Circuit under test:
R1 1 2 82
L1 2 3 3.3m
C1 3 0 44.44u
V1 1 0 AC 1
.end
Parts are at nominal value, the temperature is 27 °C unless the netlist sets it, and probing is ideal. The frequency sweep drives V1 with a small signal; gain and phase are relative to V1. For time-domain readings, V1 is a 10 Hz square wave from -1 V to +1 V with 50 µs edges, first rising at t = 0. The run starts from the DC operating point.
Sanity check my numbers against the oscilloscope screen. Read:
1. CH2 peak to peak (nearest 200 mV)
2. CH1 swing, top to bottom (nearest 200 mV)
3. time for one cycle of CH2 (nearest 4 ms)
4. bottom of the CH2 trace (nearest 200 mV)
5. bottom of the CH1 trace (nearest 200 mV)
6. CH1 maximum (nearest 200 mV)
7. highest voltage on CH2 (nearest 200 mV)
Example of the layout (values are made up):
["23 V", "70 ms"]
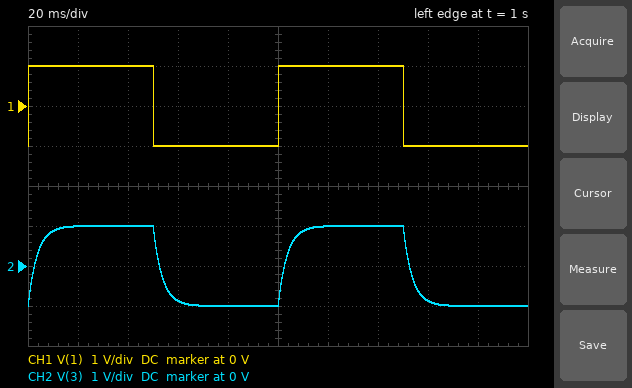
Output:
["2.0 V", "2.0 V", "100 ms", "-1.0 V", "-1.0 V", "1.0 V", "1.0 V"]
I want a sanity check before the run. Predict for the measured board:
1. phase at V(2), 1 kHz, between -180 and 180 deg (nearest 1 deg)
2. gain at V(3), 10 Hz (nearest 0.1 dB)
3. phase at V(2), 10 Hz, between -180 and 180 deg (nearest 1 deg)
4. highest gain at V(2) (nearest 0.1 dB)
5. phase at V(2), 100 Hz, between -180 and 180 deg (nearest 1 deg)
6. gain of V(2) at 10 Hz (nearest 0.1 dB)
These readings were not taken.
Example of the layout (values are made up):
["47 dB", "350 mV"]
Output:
["78 deg", "-0.2 dB", "-13 deg", "0 dB", "-68 deg", "-0.2 dB"]
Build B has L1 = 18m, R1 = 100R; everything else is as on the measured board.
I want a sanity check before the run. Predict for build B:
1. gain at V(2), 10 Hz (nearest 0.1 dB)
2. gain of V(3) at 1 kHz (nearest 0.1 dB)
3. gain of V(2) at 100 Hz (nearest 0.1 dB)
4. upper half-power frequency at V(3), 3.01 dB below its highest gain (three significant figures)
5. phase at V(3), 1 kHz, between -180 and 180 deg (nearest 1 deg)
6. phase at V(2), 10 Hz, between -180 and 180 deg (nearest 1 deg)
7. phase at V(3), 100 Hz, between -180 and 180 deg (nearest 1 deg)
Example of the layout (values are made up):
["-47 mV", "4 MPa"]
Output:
["-0.3 dB", "-32.3 dB", "-12.5 dB", "37.3 Hz", "-138 deg", "-16 deg", "-76 deg"]
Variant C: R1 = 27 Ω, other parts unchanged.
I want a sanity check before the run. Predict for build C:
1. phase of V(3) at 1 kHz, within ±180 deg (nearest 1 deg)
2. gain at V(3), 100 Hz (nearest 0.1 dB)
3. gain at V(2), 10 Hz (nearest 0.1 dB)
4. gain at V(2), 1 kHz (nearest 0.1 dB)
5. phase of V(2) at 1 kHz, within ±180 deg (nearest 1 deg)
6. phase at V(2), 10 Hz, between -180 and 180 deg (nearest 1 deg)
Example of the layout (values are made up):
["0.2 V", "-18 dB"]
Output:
["-122 deg", "-1.6 dB", "0 dB", "-5.4 dB", "58 deg", "-4 deg"]
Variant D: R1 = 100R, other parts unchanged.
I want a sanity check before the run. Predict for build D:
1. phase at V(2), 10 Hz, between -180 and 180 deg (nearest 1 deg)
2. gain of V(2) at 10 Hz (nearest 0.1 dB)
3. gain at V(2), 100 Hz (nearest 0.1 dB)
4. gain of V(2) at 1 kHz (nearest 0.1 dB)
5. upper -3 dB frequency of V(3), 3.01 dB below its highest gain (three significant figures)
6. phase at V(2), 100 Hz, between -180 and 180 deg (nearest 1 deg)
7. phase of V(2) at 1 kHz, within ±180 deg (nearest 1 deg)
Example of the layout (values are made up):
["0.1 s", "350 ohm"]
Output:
["-16 deg", "-0.3 dB", "-9.9 dB", "-15.4 dB", "36.1 Hz", "-71 deg", "80 deg"]
